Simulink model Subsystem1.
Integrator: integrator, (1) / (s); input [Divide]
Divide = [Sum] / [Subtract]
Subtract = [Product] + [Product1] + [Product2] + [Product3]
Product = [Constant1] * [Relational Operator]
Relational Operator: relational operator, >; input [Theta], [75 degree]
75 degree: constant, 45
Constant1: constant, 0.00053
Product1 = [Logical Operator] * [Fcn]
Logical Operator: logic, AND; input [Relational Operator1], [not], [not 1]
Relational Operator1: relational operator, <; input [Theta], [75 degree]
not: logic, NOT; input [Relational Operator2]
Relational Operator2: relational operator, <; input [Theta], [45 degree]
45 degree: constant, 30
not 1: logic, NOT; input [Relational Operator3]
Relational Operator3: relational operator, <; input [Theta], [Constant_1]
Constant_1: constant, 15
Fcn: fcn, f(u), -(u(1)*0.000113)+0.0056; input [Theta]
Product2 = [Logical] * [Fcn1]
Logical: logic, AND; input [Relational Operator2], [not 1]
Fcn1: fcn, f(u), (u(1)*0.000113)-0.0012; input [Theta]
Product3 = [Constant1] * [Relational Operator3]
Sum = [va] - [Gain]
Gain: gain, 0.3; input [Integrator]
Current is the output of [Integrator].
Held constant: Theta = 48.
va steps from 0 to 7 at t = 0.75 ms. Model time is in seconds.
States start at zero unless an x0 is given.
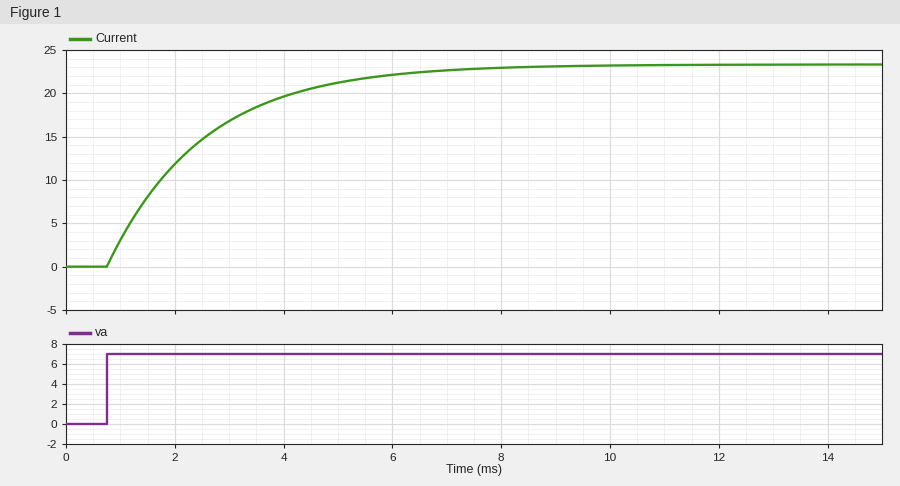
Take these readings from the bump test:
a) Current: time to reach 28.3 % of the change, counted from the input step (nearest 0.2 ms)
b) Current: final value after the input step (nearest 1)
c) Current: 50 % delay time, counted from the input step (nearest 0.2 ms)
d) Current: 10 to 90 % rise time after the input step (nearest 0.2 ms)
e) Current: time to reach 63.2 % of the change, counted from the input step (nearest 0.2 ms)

0.6 ms
23
1.2 ms
3.8 ms
1.8 ms
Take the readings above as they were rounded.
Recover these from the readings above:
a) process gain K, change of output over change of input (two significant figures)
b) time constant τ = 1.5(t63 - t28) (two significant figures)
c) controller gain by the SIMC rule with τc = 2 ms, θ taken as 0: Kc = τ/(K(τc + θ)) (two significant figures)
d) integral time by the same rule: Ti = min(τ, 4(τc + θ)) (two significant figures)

3.3
1.8 ms
0.27
1.8 ms
